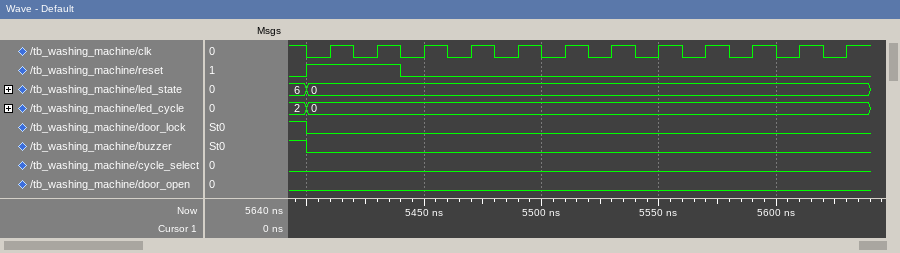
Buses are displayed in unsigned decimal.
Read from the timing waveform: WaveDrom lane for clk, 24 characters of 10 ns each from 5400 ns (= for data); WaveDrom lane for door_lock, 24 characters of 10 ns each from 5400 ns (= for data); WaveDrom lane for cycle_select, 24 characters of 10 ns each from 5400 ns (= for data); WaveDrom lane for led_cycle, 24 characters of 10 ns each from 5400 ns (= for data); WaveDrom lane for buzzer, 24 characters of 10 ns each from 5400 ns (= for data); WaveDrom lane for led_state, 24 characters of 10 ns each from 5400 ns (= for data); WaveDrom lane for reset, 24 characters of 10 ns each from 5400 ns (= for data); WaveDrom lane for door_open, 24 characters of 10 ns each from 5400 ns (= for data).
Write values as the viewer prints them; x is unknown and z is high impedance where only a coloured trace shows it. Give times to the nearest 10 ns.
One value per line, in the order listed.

{name: 'clk', wave: '010101010101010101010101'}
{name: 'door_lock', wave: '0.......................'}
{name: 'cycle_select', wave: '0.......................'}
{name: 'led_cycle', wave: '=.......................', data: '0'}
{name: 'buzzer', wave: '0.......................'}
{name: 'led_state', wave: '=.......................', data: '0'}
{name: 'reset', wave: '1...0...................'}
{name: 'door_open', wave: '0.......................'}
